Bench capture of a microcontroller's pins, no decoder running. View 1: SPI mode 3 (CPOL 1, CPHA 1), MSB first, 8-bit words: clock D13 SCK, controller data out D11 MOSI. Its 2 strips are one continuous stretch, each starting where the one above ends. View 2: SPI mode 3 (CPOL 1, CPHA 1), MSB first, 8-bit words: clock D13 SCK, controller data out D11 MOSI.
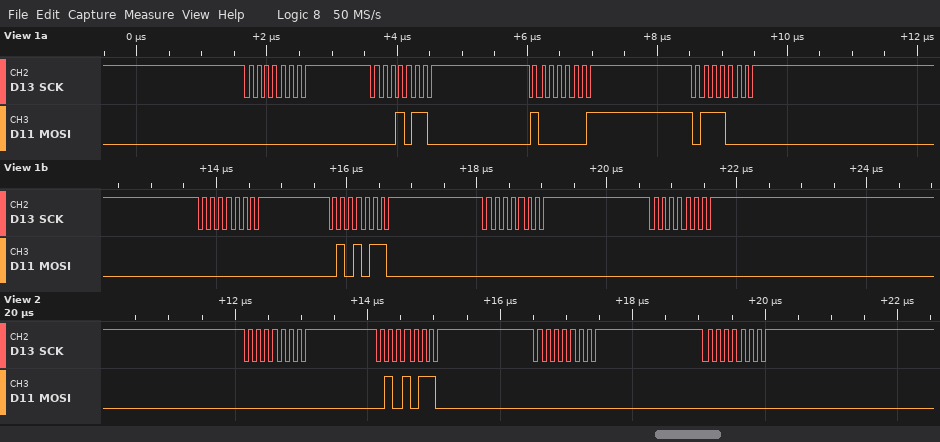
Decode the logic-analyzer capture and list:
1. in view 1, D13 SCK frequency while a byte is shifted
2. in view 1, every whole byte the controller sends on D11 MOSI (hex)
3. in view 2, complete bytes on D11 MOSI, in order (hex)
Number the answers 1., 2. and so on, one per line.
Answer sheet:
1. 8 MHz
2. 00 16 81 70 00 56 00 00
3. 00 56 00 00
